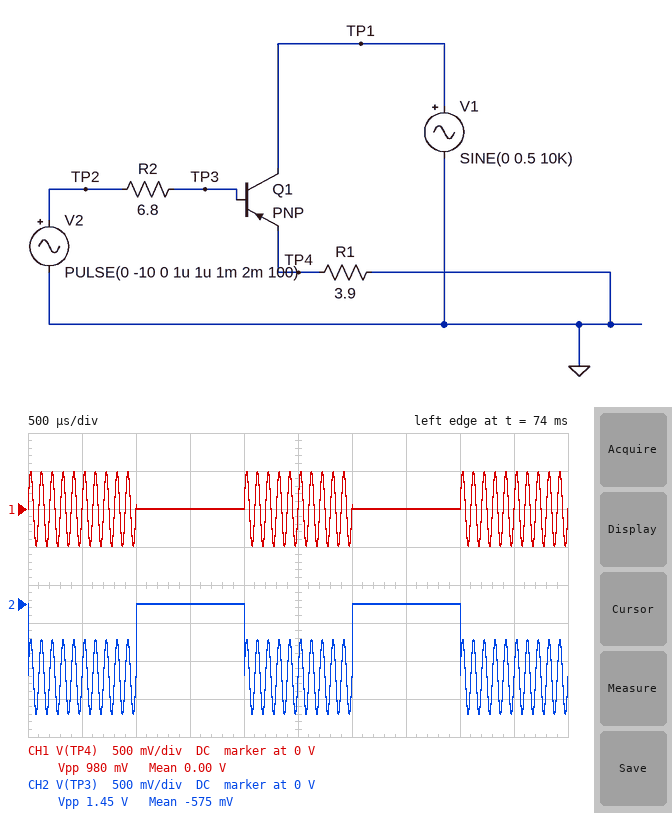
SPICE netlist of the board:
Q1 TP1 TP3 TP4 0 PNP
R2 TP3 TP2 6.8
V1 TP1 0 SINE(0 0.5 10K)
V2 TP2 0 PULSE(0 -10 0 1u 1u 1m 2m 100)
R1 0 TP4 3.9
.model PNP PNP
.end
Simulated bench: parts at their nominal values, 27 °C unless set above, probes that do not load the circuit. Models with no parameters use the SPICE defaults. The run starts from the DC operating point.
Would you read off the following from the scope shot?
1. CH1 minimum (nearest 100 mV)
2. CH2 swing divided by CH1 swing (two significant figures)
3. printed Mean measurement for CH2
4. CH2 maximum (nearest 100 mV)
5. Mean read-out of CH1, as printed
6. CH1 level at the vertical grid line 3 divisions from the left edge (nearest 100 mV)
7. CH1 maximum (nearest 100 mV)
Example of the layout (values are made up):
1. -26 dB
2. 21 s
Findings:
1. -500 mV
2. 1.5
3. -575 mV
4. 0 V
5. 0.00 V
6. 0 V
7. 500 mV
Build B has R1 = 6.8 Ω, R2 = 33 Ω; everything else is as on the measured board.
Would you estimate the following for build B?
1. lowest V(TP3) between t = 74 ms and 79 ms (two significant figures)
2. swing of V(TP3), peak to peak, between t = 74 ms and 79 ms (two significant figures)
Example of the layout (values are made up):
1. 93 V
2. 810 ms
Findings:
1. -1.4 V
2. 1.4 V
